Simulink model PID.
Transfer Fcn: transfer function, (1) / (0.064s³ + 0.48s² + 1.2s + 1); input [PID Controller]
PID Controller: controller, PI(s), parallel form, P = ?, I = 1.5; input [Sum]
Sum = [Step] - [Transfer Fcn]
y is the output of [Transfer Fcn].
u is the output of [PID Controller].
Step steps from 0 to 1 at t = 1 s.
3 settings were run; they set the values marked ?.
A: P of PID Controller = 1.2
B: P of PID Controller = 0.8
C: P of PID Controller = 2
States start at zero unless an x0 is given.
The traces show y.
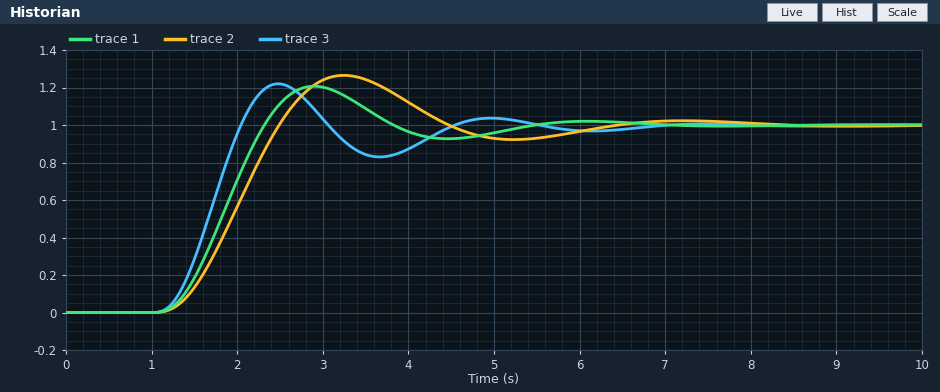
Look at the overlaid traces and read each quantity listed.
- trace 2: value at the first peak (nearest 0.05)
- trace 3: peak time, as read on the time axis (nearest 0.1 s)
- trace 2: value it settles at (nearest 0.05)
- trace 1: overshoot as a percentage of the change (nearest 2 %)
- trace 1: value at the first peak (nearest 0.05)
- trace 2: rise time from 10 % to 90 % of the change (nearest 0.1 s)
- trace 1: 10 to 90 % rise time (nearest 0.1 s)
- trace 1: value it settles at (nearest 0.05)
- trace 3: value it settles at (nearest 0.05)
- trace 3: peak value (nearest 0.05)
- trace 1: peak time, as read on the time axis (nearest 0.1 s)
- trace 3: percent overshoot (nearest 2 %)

1.25
2.5 s
1.00
20 %
1.20
0.9 s
0.8 s
1.00
1.00
1.20
2.9 s
22 %
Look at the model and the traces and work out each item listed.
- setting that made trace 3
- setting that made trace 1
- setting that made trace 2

C
A
B
